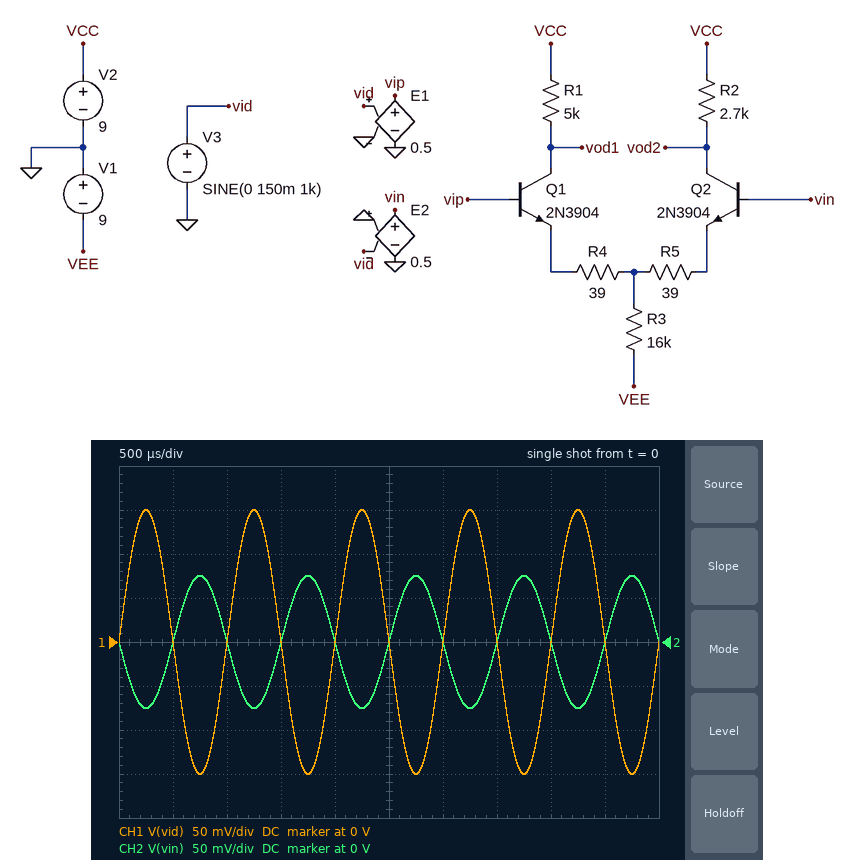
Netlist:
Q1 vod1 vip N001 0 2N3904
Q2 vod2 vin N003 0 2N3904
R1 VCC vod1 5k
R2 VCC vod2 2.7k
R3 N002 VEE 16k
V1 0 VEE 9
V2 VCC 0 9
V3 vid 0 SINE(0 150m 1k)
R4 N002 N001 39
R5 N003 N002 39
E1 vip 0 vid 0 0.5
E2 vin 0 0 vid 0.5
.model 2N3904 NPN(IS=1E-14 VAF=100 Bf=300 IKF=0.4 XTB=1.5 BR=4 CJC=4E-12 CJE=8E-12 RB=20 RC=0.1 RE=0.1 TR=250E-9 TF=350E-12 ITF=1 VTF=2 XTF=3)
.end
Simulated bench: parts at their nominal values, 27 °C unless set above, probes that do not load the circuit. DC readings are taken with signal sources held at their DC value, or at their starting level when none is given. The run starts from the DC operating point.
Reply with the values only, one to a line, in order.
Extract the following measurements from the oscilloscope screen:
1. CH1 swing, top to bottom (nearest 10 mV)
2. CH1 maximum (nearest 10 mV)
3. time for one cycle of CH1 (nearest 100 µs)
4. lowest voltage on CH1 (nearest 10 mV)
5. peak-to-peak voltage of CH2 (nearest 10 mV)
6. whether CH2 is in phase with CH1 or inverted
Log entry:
300 mV
150 mV
1.0 ms
-150 mV
150 mV
inverted
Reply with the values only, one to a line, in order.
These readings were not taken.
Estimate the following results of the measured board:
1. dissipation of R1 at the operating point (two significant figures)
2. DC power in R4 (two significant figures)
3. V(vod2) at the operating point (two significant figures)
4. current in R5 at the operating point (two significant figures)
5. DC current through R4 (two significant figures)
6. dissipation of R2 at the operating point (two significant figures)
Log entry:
340 µW
2.7 µW
8.3 V
260 µA
260 µA
180 µW
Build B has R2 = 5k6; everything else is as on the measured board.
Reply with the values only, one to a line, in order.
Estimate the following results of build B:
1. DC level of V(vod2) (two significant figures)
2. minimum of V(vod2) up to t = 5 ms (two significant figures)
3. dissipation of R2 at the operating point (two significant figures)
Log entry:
7.5 V
6.1 V
380 µW
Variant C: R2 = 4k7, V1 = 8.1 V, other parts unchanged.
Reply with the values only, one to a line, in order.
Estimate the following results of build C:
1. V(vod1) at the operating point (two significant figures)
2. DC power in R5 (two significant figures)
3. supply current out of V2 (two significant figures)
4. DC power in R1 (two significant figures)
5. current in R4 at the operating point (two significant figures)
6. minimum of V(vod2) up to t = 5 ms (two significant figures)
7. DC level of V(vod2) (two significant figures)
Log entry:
7.8 V
2.1 µW
470 µA
270 µW
230 µA
6.8 V
7.9 V
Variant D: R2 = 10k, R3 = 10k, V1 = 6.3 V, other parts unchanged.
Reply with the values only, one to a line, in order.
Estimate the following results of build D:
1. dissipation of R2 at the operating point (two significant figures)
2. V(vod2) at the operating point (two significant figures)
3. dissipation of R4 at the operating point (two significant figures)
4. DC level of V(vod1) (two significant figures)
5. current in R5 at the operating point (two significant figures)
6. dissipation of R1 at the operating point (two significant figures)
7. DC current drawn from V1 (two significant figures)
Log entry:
790 µW
6.2 V
3.2 µW
7.6 V
280 µA
400 µW
570 µA
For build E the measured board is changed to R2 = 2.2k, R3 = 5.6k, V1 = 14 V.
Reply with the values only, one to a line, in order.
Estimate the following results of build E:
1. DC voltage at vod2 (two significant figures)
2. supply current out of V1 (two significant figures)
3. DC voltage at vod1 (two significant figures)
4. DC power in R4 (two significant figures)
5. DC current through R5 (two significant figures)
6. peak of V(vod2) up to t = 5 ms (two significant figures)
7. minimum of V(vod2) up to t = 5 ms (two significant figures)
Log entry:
6.4 V
2.4 mA
3.1 V
54 µW
1.2 mA
8.5 V
4.1 V
